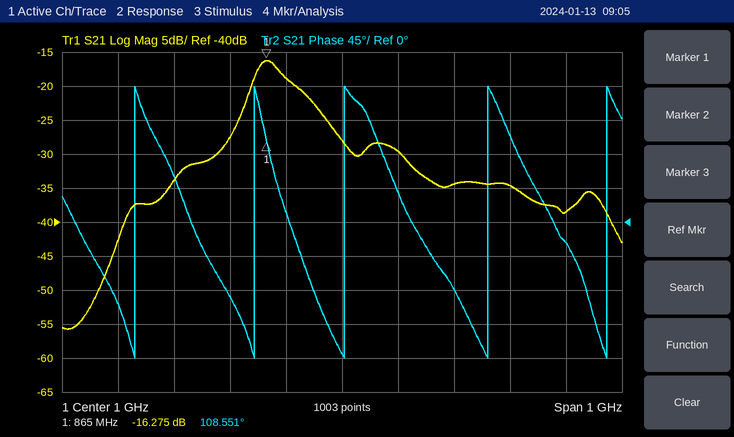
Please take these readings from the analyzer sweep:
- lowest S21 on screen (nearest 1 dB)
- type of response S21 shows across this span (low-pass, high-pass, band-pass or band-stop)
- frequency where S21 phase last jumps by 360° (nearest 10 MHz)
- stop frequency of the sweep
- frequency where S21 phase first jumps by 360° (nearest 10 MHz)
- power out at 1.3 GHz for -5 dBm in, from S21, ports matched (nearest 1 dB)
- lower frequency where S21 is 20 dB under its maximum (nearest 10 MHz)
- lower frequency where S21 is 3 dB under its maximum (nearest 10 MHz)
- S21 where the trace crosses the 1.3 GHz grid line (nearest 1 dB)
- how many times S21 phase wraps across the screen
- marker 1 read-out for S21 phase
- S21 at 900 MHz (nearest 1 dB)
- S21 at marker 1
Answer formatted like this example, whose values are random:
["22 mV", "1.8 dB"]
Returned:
["-56 dB", "band-pass", "1.47 GHz", "1.5 GHz", "630 MHz", "-40 dBm", "680 MHz", "840 MHz", "-35 dB", "5", "108.551°", "-19 dB", "-16.275 dB"]
